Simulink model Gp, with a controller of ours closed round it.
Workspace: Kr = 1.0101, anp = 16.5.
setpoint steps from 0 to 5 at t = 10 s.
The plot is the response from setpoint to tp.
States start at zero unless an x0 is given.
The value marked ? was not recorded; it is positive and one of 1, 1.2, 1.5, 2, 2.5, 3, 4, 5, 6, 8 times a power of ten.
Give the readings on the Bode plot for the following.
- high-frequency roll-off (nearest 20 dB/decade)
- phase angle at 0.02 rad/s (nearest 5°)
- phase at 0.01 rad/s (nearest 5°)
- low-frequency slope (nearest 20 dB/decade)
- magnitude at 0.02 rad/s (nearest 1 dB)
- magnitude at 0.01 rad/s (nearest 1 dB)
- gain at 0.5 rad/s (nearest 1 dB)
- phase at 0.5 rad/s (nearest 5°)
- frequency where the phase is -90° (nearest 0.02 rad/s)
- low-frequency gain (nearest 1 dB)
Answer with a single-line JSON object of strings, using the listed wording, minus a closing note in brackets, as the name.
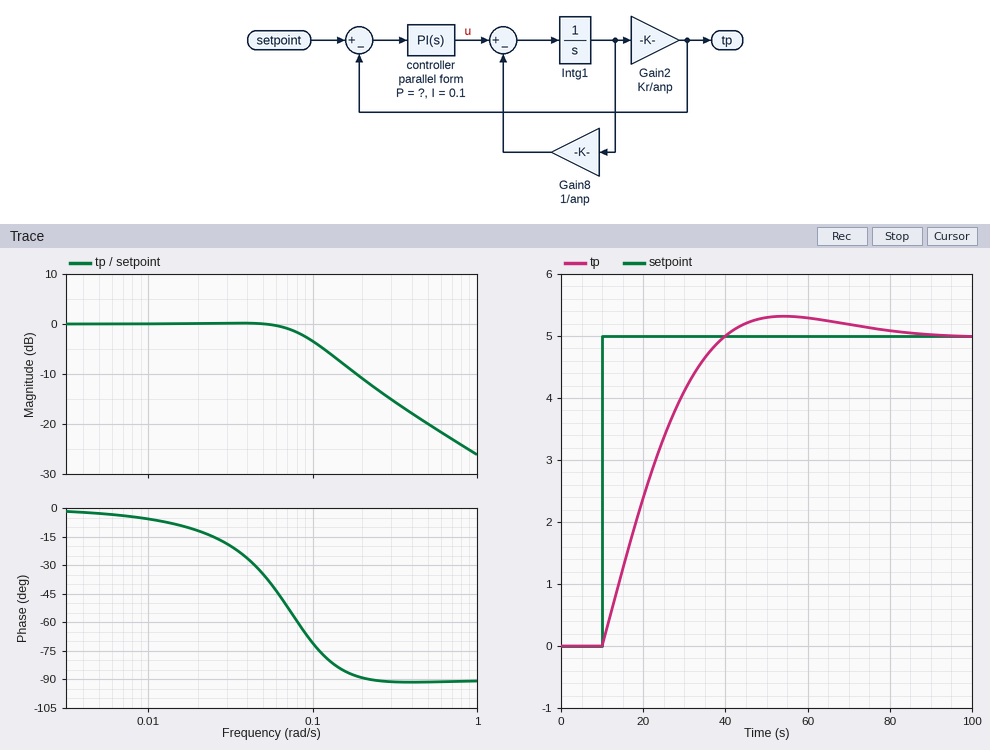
{"high-frequency roll-off": "-20 dB/decade", "phase angle at 0.02 rad/s": "-10°", "phase at 0.01 rad/s": "-5°", "low-frequency slope": "0 dB/decade", "magnitude at 0.02 rad/s": "0 dB", "magnitude at 0.01 rad/s": "0 dB", "gain at 0.5 rad/s": "-20 dB", "phase at 0.5 rad/s": "-90°", "frequency where the phase is -90°": "0.22 rad/s", "low-frequency gain": "0 dB"}
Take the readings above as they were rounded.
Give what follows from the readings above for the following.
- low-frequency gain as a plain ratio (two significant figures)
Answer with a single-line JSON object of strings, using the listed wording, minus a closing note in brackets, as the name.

{"low-frequency gain as a plain ratio": "1.0"}
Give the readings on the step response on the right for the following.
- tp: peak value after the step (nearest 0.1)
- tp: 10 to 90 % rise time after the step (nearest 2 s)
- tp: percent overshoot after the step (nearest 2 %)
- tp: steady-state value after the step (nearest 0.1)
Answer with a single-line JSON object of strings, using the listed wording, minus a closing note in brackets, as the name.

{"tp: peak value after the step": "5.3", "tp: 10 to 90 % rise time after the step": "22 s", "tp: percent overshoot after the step": "6 %", "tp: steady-state value after the step": "5.0"}
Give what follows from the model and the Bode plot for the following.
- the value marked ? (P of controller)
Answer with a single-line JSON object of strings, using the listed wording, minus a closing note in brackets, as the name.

{"the value marked ?": "0.8"}
